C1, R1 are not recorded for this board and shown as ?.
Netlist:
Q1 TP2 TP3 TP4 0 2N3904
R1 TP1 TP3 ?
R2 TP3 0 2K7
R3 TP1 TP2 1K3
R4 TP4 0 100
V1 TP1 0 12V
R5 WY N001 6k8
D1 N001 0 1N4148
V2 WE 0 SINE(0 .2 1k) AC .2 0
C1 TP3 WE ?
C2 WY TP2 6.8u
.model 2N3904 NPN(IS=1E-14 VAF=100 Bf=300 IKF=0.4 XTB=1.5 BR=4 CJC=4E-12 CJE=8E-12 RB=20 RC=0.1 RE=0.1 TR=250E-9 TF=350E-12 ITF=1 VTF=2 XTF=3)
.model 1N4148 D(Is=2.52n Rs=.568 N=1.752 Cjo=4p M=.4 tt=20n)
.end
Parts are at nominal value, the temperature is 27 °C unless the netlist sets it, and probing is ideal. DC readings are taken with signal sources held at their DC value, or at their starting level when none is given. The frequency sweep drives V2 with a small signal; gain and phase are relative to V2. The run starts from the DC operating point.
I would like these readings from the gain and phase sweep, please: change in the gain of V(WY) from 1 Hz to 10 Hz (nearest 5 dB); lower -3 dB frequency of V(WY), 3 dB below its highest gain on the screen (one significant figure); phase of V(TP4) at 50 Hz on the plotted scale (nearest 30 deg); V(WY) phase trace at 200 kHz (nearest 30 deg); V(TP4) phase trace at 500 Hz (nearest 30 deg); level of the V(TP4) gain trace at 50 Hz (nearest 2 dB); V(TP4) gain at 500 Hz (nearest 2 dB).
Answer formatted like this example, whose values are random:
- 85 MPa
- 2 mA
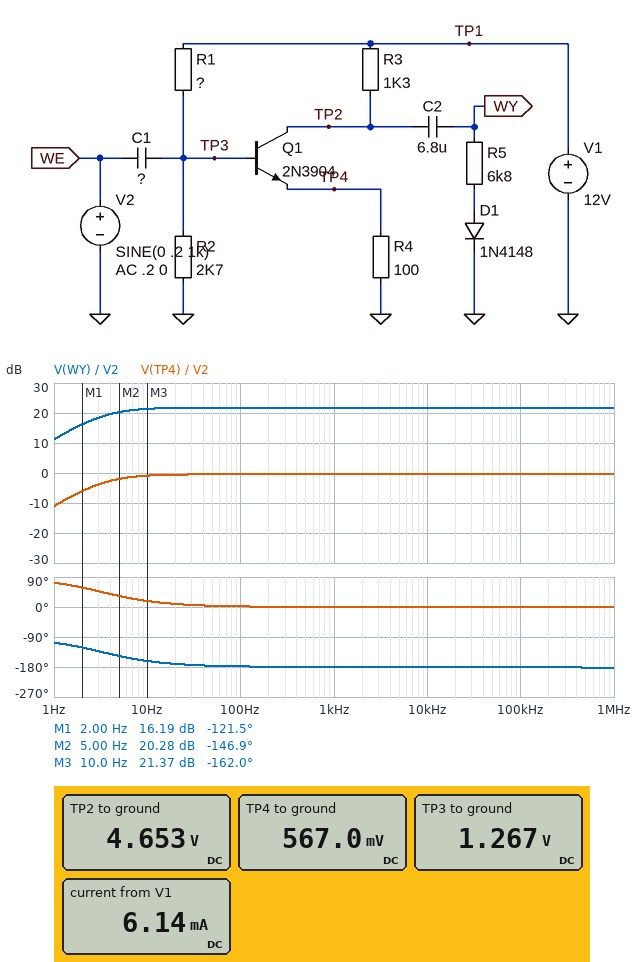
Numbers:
- 10 dB
- 3 Hz
- 0 deg
- -180 deg
- 0 deg
- 0 dB
- 0 dB
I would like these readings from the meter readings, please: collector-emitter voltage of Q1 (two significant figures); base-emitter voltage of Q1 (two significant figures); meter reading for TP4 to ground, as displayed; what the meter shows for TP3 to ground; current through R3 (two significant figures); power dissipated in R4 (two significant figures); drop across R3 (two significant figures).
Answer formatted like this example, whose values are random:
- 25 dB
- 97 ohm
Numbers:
- 4.1 V
- 700 mV
- 567.0 mV
- 1.267 V
- 5.7 mA
- 3.2 mW
- 7.3 V
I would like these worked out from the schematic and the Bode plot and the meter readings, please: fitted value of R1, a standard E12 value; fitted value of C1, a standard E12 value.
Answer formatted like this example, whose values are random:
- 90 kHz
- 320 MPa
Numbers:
- 22 kΩ
- 22 µF
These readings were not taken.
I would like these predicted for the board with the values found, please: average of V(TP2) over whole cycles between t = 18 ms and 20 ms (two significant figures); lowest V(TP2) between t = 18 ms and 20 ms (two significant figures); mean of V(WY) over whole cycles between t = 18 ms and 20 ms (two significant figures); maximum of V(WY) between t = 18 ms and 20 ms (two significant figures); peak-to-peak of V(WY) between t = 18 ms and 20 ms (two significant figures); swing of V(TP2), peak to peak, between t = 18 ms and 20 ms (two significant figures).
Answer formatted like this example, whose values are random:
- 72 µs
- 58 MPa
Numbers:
- 4.6 V
- 2.2 V
- -250 mV
- 2.0 V
- 4.6 V
- 4.6 V
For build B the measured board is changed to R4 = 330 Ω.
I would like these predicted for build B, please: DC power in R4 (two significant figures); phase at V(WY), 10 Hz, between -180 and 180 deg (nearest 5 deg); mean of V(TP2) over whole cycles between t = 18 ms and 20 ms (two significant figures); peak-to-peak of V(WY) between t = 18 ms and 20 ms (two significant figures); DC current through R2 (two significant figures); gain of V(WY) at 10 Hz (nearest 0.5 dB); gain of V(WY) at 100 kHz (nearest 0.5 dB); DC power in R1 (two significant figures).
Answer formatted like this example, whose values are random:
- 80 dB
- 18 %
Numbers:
- 1.2 mW
- -165 deg
- 9.5 V
- 1.5 V
- 480 µA
- 11.0 dB
- 11.5 dB
- 5.2 mW
